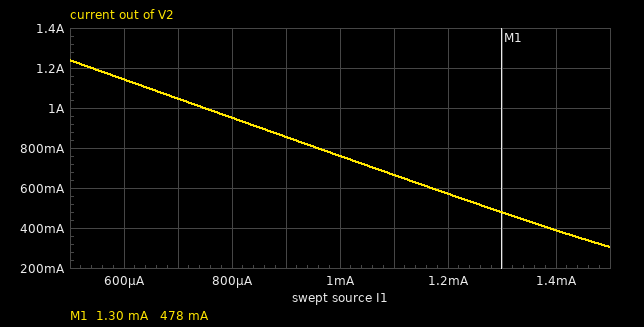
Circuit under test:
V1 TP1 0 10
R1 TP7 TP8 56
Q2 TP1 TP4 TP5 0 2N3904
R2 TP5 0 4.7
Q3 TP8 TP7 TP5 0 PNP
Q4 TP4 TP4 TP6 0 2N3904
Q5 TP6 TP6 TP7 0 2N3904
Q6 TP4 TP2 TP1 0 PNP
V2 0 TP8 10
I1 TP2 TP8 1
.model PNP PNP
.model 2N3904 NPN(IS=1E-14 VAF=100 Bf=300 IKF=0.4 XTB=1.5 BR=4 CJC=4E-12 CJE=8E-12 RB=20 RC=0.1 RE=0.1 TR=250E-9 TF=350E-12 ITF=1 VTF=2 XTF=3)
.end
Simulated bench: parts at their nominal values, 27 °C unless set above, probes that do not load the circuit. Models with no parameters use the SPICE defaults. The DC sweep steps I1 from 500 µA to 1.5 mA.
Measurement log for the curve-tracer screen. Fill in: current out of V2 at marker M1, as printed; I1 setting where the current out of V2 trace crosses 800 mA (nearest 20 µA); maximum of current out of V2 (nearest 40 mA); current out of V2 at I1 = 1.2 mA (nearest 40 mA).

478 mA
960 µA
1.24 A
560 mA
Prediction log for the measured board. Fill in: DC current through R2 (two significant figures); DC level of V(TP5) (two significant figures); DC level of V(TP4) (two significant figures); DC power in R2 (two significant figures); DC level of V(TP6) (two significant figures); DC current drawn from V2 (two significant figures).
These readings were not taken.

1.8 A
8.3 V
10 V
15 W
9.1 V
1.3 A
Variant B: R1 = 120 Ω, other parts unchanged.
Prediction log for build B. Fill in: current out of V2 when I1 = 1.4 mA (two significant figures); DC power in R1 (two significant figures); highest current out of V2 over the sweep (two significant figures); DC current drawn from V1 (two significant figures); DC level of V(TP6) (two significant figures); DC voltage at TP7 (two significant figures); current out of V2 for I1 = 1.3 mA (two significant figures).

130 mA
2.8 W
570 mA
2.9 A
9.2 V
8.3 V
120 mA
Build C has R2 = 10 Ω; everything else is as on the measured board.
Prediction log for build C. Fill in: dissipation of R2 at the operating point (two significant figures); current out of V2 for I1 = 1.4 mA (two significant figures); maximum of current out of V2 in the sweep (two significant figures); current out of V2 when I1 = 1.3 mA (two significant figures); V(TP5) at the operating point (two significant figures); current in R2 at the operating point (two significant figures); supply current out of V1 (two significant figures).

7.8 W
280 mA
640 mA
310 mA
8.8 V
880 mA
2.2 A
